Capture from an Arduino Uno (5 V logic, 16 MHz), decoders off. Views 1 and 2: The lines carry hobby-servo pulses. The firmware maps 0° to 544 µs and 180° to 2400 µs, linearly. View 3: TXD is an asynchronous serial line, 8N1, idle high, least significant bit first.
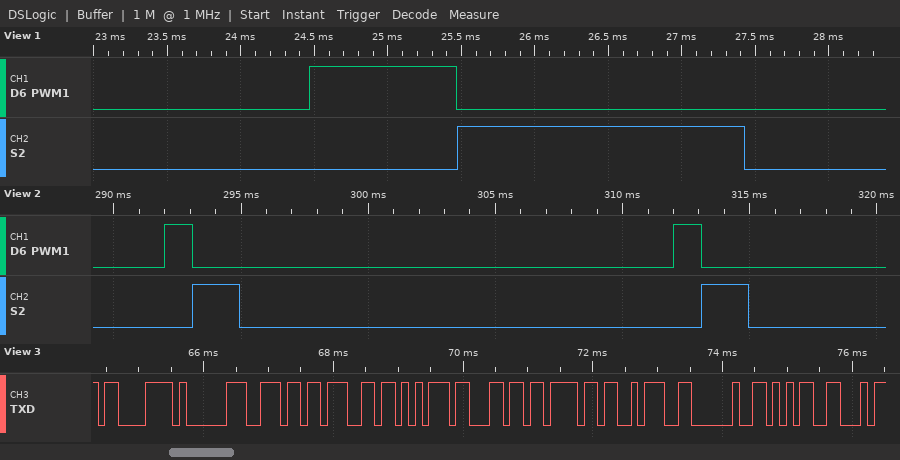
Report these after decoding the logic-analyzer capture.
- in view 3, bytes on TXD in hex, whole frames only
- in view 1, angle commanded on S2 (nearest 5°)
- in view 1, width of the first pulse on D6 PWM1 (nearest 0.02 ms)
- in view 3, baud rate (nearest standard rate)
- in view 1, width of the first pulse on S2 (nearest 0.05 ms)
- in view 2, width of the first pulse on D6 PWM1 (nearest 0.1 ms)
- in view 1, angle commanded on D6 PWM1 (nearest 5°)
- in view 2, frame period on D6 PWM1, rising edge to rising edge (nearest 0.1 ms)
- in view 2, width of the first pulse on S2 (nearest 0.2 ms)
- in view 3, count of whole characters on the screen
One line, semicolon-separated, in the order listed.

0xC3 0x81 0x6E 0x67 0x75 0x6C 0x6F 0x3A 0x20 0x35; 135°; 1.00 ms; 9600 baud; 1.95 ms; 1.1 ms; 45°; 20.0 ms; 1.8 ms; 10
